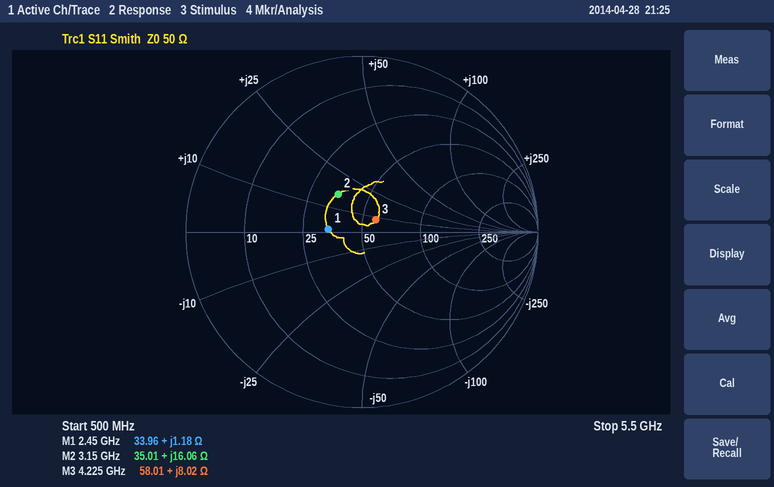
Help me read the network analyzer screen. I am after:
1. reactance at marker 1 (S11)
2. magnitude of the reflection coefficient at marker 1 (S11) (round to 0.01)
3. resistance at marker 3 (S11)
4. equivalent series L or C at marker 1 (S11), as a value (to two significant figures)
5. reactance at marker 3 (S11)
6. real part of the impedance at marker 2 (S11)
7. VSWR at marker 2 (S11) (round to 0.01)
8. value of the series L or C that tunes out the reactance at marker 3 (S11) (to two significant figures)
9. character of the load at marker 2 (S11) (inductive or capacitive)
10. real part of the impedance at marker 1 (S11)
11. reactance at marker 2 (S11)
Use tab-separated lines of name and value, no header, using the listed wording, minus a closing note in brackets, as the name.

reactance at marker 1	+1.18 Ω
magnitude of the reflection coefficient at marker 1 (S11)	0.19
resistance at marker 3	58.01 Ω
equivalent series L or C at marker 1 (S11), as a value	77 pH
reactance at marker 3	+8.02 Ω
real part of the impedance at marker 2	35.01 Ω
VSWR at marker 2 (S11)	1.68
value of the series L or C that tunes out the reactance at marker 3 (S11)	4.7 pF
character of the load at marker 2 (S11)	inductive
real part of the impedance at marker 1	33.96 Ω
reactance at marker 2	+16.06 Ω
